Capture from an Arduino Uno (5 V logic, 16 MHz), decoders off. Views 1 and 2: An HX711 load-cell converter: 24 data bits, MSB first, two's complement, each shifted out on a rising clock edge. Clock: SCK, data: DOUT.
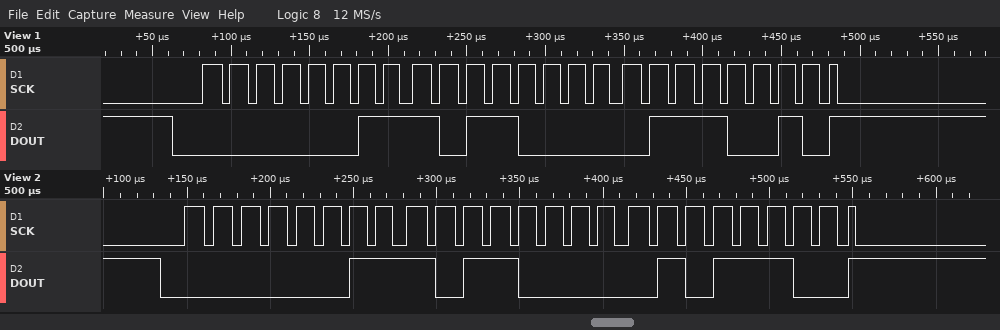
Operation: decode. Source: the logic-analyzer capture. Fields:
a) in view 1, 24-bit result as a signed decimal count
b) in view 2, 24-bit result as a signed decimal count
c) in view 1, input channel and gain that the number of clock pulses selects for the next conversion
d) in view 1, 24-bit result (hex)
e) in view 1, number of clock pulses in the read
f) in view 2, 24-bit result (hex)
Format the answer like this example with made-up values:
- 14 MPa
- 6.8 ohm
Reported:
- 241778
- 241756
- channel A, gain 128
- 0x03B072
- 25
- 0x03B05C
